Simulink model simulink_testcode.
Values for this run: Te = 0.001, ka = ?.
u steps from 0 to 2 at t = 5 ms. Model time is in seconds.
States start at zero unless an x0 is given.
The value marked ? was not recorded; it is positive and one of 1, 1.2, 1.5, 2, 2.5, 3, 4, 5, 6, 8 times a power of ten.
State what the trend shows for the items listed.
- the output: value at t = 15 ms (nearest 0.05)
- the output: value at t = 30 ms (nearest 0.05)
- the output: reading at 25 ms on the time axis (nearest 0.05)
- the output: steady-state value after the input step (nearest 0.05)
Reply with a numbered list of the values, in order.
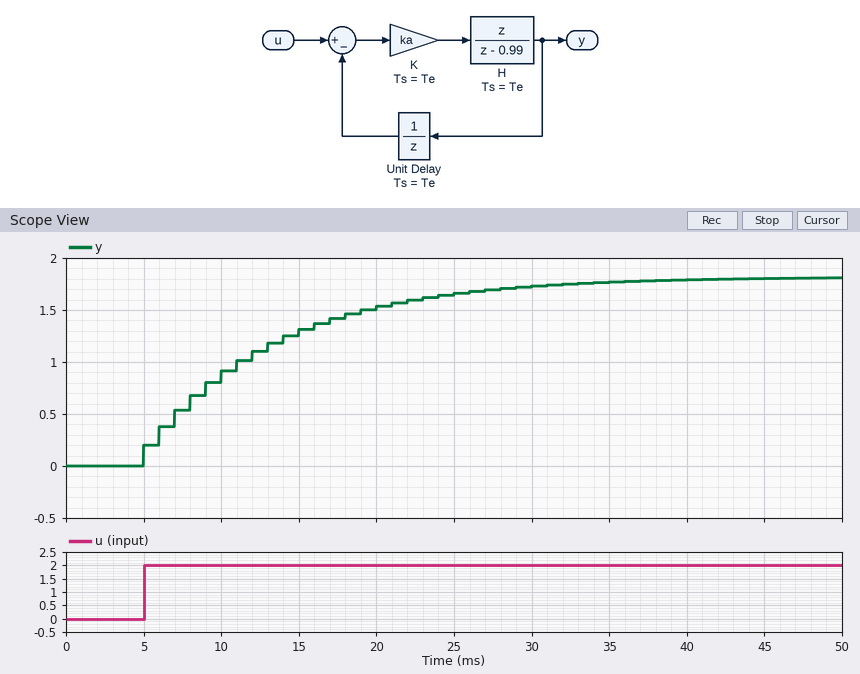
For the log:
1. 1.30
2. 1.75
3. 1.65
4. 1.80
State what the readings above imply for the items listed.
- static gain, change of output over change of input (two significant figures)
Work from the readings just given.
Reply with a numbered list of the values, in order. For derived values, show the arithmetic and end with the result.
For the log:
1. (1.8 - 0) / (2 - 0) = 0.90
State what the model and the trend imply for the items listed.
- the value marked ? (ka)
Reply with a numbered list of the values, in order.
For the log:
1. 0.1
